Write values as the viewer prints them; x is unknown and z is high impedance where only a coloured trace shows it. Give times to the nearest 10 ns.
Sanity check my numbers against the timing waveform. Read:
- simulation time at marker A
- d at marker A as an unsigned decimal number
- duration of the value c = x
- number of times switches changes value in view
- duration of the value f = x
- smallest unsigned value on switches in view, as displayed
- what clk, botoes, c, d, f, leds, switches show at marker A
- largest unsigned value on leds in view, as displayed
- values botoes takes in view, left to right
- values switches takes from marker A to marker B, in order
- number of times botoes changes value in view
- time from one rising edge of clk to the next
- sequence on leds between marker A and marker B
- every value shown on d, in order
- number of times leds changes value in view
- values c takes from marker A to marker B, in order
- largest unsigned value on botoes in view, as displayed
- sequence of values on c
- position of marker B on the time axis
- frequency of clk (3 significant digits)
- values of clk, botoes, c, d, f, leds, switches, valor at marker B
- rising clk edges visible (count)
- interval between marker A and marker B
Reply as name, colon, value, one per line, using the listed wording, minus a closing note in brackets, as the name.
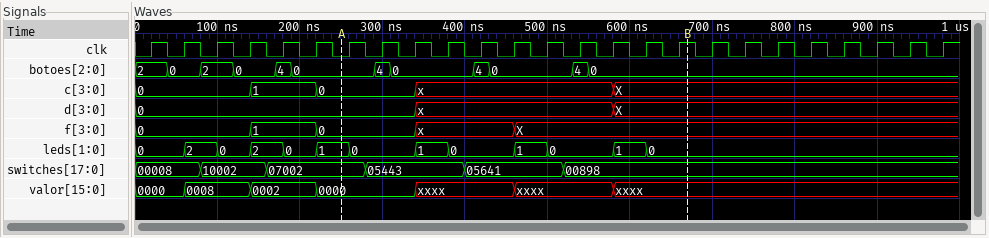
simulation time at marker A: 250 ns
d at marker A as an unsigned decimal number: 0
duration of the value c = x: 240 ns
number of times switches changes value in view: 5
duration of the value f = x: 120 ns
smallest unsigned value on switches in view, as displayed: 00008
what clk, botoes, c, d, f, leds, switches show at marker A: clk=0, botoes=0, c=0, d=0, f=0, leds=1, switches=07002
largest unsigned value on leds in view, as displayed: 2
values botoes takes in view, left to right: 2, 0, 2, 0, 4, 0, 4, 0, 4, 0, 4, 0
values switches takes from marker A to marker B, in order: 07002, 05443, 05641, 00898
number of times botoes changes value in view: 11
time from one rising edge of clk to the next: 40 ns
sequence on leds between marker A and marker B: 1, 0, 1, 0, 1, 0, 1, 0
every value shown on d, in order: 0, x, X
number of times leds changes value in view: 12
values c takes from marker A to marker B, in order: 0, x, X
largest unsigned value on botoes in view, as displayed: 4
sequence of values on c: 0, 1, 0, x, X
position of marker B on the time axis: 670 ns
frequency of clk: 25.0 MHz
values of clk, botoes, c, d, f, leds, switches, valor at marker B: clk=1, botoes=0, c=X, d=X, f=X, leds=0, switches=00898, valor=xxxx
rising clk edges visible: 25
interval between marker A and marker B: 420 ns
